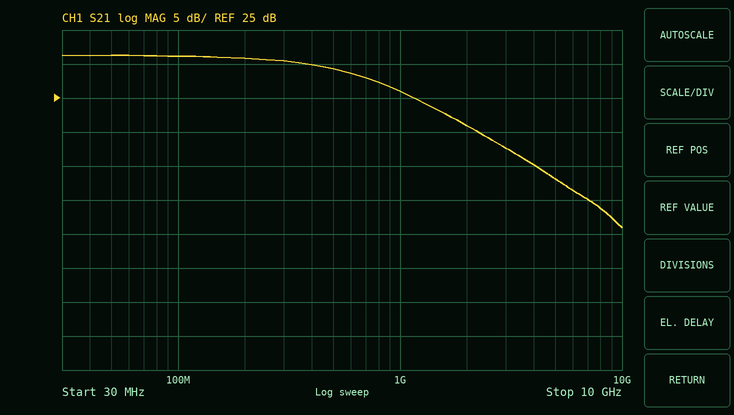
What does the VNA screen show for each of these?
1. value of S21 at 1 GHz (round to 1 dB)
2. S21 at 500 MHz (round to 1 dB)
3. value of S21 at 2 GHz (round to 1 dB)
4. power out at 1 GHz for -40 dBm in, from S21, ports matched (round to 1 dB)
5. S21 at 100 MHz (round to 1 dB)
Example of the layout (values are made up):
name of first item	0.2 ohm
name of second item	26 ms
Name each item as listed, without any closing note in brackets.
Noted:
value of S21 at 1 GHz	26 dB
S21 at 500 MHz	29 dB
value of S21 at 2 GHz	21 dB
power out at 1 GHz for -40 dBm in, from S21, ports matched	-14 dBm
S21 at 100 MHz	31 dB
